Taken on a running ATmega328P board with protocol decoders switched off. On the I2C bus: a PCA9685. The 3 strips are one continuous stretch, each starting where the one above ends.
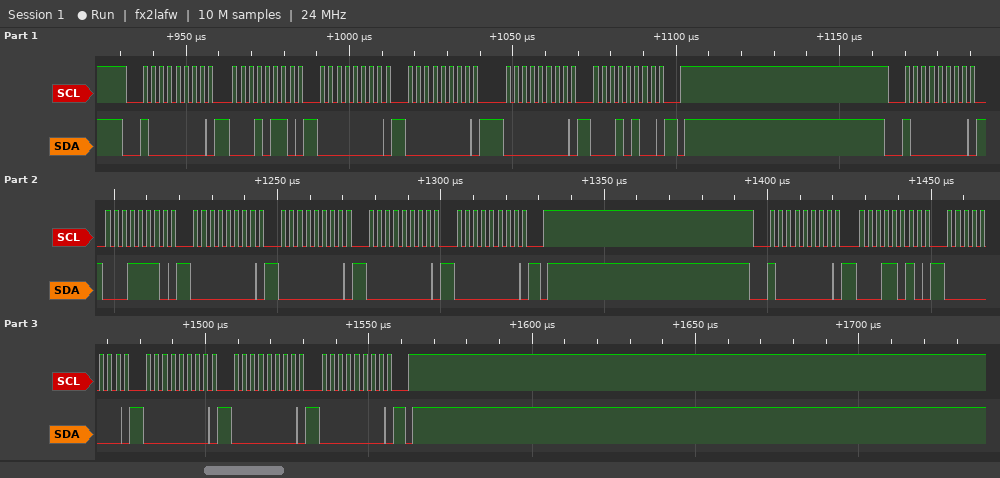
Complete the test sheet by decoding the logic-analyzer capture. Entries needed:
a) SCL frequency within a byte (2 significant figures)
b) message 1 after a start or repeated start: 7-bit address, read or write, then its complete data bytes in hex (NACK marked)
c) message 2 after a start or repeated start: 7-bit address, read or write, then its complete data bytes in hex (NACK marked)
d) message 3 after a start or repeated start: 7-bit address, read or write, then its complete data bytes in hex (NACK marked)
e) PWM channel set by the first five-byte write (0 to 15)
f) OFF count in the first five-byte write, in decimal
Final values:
400 kHz
0x40 write: 16 00 00 00 14
0x40 write: 1E 00 00 00 00
0x40 write: 1A 00 00 00 00
4
5120
